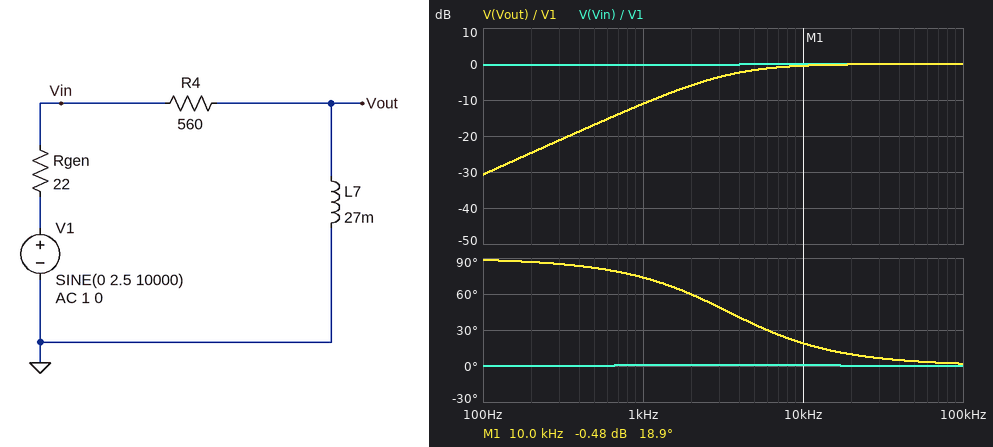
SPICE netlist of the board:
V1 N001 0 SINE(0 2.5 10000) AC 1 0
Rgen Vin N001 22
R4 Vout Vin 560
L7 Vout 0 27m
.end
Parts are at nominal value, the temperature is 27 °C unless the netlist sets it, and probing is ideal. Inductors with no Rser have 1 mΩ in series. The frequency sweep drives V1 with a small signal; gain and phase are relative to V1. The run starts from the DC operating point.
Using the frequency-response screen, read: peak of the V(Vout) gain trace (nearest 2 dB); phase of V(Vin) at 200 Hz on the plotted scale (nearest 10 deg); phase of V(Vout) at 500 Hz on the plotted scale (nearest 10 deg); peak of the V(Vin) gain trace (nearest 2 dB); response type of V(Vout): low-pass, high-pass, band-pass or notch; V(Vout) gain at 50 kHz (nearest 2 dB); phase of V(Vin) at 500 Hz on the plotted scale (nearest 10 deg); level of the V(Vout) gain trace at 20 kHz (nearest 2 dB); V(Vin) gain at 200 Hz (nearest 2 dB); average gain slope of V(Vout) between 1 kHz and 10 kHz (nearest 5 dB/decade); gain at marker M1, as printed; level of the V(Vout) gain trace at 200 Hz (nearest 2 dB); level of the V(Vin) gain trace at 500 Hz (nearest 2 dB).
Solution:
0 dB
0 deg
80 deg
0 dB
high-pass
0 dB
0 deg
0 dB
0 dB
10 dB/decade
-0.48 dB
-24 dB
0 dB
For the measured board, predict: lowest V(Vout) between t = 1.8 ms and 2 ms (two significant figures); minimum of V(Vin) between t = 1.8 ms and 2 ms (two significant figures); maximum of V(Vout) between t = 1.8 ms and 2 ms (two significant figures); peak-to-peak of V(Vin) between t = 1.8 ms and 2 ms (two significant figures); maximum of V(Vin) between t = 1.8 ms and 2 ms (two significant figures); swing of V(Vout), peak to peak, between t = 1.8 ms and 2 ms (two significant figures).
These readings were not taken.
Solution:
-2.4 V
-2.5 V
2.4 V
5.0 V
2.5 V
4.7 V
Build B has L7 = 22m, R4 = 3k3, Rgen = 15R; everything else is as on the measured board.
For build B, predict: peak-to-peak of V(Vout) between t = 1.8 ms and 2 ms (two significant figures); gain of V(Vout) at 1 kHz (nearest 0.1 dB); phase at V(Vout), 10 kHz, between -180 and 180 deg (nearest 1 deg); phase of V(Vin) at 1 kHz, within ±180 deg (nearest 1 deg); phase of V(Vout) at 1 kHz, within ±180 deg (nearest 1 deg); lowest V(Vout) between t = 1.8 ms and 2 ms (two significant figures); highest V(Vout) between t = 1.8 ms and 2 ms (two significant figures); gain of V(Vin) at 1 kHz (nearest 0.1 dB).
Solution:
1.9 V
-27.6 dB
67 deg
0 deg
88 deg
-960 mV
960 mV
0 dB
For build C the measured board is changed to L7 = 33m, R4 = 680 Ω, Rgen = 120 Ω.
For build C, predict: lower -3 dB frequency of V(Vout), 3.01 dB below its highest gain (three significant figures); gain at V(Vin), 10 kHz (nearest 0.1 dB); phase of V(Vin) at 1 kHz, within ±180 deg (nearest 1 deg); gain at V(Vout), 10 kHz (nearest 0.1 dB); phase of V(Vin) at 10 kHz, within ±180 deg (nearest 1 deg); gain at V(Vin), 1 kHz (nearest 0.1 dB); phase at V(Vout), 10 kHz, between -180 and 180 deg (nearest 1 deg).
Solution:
3.86 kHz
-0.2 dB
2 deg
-0.6 dB
3 deg
-1.3 dB
21 deg
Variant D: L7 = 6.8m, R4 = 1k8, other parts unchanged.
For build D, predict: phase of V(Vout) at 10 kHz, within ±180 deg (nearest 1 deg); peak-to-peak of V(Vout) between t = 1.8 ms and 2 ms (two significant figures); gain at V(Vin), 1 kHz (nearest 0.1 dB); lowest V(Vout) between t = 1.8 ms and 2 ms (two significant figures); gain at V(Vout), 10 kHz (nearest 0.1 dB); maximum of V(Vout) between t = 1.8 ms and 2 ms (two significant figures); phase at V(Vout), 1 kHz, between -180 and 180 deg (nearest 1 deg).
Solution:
77 deg
1.1 V
-0.1 dB
-570 mV
-12.8 dB
570 mV
89 deg
